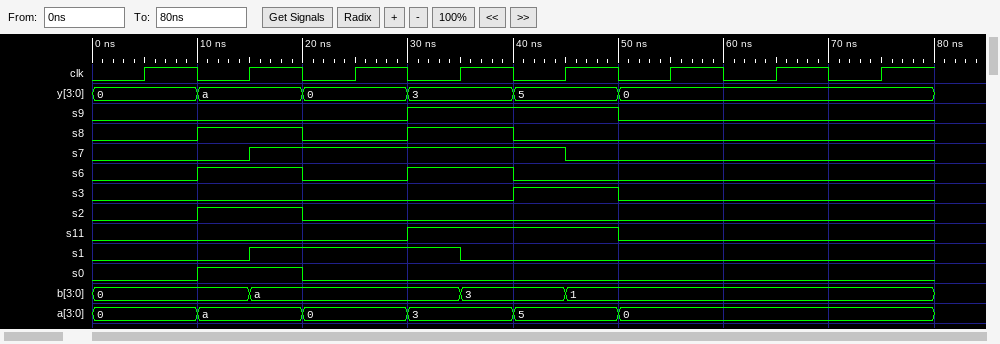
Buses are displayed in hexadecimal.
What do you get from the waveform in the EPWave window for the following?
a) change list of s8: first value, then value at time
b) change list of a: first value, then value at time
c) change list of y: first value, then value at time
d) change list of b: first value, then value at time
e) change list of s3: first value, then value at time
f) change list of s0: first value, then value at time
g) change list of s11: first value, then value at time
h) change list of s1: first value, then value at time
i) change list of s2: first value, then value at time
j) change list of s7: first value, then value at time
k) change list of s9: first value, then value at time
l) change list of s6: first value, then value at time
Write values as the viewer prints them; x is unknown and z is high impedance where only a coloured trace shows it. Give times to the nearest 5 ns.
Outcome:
0, 1 at 10 ns, 0 at 20 ns, 1 at 30 ns, 0 at 40 ns
0, a at 10 ns, 0 at 20 ns, 3 at 30 ns, 5 at 40 ns, 0 at 50 ns
0, a at 10 ns, 0 at 20 ns, 3 at 30 ns, 5 at 40 ns, 0 at 50 ns
0, a at 15 ns, 3 at 35 ns, 1 at 45 ns
0, 1 at 40 ns, 0 at 50 ns
0, 1 at 10 ns, 0 at 20 ns
0, 1 at 30 ns, 0 at 50 ns
0, 1 at 15 ns, 0 at 35 ns
0, 1 at 10 ns, 0 at 20 ns
0, 1 at 15 ns, 0 at 45 ns
0, 1 at 30 ns, 0 at 50 ns
0, 1 at 10 ns, 0 at 20 ns, 1 at 30 ns, 0 at 40 ns
